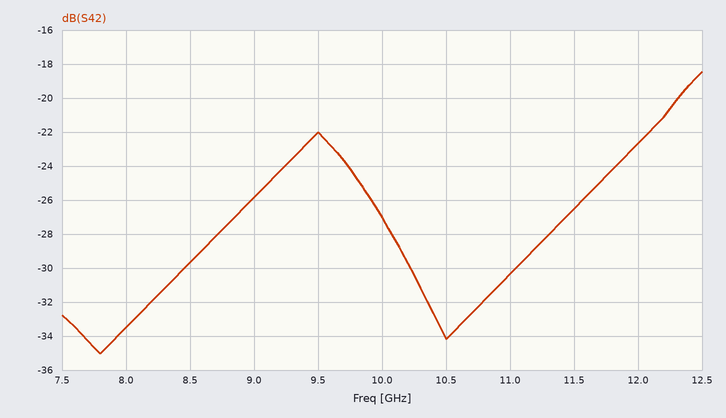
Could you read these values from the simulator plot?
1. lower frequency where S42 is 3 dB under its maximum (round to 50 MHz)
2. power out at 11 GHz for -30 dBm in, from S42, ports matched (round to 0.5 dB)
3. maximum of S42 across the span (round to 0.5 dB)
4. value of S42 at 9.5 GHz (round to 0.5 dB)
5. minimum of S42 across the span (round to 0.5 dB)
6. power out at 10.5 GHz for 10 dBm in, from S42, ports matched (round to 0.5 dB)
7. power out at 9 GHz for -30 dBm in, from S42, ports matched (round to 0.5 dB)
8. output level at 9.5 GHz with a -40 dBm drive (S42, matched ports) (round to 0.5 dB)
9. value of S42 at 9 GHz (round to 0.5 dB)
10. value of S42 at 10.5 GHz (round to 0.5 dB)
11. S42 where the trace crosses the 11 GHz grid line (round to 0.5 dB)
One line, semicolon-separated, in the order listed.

12.15 GHz; -60.5 dBm; -18.5 dB; -22.0 dB; -35.0 dB; -24.0 dBm; -56.0 dBm; -62.0 dBm; -26.0 dB; -34.0 dB; -30.5 dB
